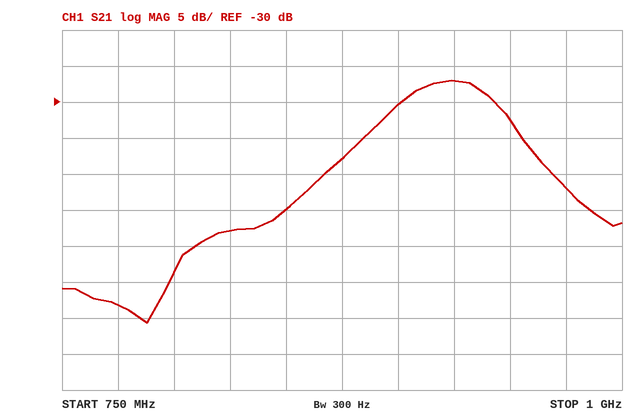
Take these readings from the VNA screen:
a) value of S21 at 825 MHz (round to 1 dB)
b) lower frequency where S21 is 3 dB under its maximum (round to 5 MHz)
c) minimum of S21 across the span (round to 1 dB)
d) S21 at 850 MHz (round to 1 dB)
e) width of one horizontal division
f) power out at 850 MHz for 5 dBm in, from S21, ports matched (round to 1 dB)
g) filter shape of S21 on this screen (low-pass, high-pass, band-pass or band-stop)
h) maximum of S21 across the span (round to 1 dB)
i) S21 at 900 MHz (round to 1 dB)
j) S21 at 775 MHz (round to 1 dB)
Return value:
-48 dB
900 MHz
-61 dB
-45 dB
25 MHz
-40 dBm
band-pass
-27 dB
-30 dB
-58 dB
